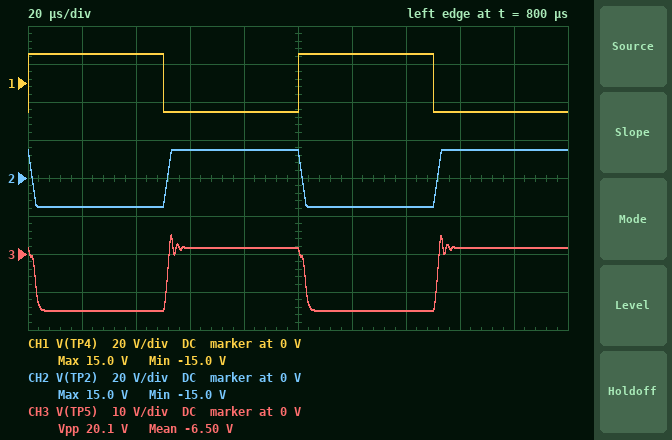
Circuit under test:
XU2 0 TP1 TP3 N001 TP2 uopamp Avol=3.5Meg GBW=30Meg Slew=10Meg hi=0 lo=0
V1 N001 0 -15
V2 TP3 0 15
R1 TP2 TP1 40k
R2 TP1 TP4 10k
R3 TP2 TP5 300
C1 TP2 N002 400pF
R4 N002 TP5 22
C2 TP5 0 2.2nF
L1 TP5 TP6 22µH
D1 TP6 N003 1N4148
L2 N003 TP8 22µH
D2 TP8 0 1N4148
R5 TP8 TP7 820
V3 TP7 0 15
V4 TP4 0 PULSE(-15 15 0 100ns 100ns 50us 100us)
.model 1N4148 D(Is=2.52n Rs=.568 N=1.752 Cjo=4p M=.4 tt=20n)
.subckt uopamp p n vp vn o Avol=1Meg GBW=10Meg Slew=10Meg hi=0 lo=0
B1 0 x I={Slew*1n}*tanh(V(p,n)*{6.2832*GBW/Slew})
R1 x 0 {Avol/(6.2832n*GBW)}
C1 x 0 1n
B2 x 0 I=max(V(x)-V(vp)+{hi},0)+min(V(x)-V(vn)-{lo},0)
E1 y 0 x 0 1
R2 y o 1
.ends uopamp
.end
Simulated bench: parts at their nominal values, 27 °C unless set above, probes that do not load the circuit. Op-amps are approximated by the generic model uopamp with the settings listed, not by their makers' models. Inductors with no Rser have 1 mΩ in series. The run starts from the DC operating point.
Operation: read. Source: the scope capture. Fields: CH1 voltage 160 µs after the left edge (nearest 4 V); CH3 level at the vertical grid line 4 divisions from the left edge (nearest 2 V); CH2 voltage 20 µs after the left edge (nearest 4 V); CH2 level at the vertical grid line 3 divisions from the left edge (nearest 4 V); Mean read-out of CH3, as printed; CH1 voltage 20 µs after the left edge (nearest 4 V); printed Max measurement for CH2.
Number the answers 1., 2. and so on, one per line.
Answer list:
1. -16 V
2. 2 V
3. -16 V
4. 16 V
5. -6.50 V
6. 16 V
7. 15.0 V
